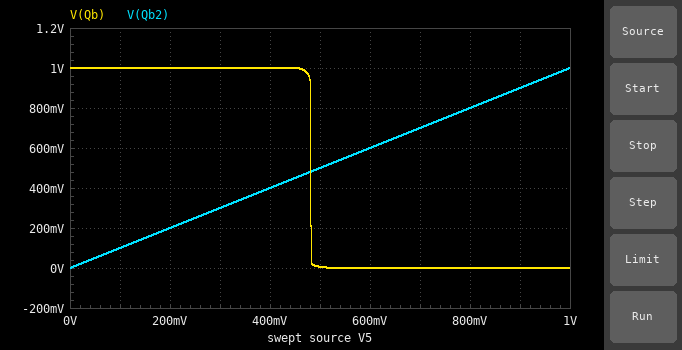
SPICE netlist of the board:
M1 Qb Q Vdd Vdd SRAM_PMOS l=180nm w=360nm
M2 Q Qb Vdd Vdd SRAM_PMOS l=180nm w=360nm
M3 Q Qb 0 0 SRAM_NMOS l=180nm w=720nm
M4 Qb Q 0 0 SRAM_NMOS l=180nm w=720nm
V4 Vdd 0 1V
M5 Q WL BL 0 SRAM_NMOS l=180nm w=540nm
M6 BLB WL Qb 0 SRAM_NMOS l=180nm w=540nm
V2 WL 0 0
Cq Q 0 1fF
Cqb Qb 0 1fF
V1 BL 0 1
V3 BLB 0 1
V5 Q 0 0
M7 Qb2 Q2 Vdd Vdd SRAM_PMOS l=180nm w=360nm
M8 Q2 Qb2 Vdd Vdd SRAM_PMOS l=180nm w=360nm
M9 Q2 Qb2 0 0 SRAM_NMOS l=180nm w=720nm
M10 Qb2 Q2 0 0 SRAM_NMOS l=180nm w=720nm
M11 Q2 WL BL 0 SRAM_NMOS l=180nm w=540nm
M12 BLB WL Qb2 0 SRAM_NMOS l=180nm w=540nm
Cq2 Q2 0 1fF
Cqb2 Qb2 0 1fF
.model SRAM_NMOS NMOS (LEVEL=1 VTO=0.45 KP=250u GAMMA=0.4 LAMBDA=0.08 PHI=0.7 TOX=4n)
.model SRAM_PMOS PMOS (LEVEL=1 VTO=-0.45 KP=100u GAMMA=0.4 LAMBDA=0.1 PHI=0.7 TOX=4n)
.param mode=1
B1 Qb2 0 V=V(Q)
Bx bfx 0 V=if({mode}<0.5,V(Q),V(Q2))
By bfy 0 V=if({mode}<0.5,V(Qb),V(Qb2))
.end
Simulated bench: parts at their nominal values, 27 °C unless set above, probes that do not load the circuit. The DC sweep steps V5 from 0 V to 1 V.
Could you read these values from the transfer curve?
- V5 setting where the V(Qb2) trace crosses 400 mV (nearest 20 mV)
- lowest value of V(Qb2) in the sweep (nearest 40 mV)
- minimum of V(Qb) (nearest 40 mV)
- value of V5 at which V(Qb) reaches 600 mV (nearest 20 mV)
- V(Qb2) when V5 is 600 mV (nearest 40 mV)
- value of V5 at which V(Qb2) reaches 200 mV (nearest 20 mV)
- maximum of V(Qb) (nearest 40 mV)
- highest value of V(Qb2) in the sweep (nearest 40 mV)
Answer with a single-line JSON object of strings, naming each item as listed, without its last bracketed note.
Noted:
{"V5 setting where the V(Qb2) trace crosses 400 mV": "400 mV", "lowest value of V(Qb2) in the sweep": "0 V", "minimum of V(Qb)": "0 V", "value of V5 at which V(Qb) reaches 600 mV": "480 mV", "V(Qb2) when V5 is 600 mV": "600 mV", "value of V5 at which V(Qb2) reaches 200 mV": "200 mV", "maximum of V(Qb)": "1.00 V", "highest value of V(Qb2) in the sweep": "1.00 V"}
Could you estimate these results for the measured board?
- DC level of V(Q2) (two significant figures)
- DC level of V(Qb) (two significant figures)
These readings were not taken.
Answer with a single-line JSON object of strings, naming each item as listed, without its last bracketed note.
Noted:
{"DC level of V(Q2)": "1.0 V", "DC level of V(Qb)": "1.0 V"}
